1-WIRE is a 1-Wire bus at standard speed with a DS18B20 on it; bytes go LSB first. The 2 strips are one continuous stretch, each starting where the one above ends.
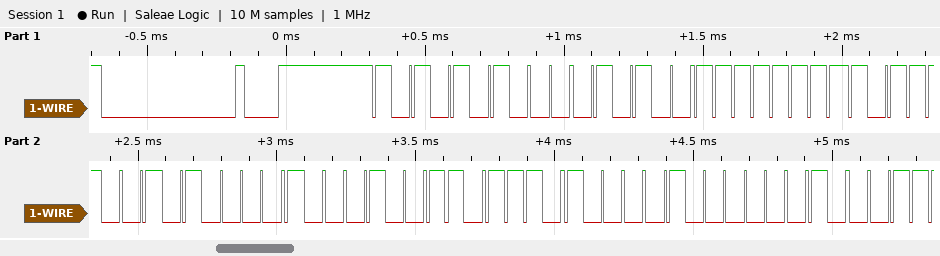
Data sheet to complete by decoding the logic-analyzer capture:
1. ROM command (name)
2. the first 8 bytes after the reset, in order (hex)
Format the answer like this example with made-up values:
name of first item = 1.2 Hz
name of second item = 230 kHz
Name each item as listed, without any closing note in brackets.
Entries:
ROM command = Match ROM
the first 8 bytes after the reset, in order = 55 28 FF 9D 42 64 17 02
